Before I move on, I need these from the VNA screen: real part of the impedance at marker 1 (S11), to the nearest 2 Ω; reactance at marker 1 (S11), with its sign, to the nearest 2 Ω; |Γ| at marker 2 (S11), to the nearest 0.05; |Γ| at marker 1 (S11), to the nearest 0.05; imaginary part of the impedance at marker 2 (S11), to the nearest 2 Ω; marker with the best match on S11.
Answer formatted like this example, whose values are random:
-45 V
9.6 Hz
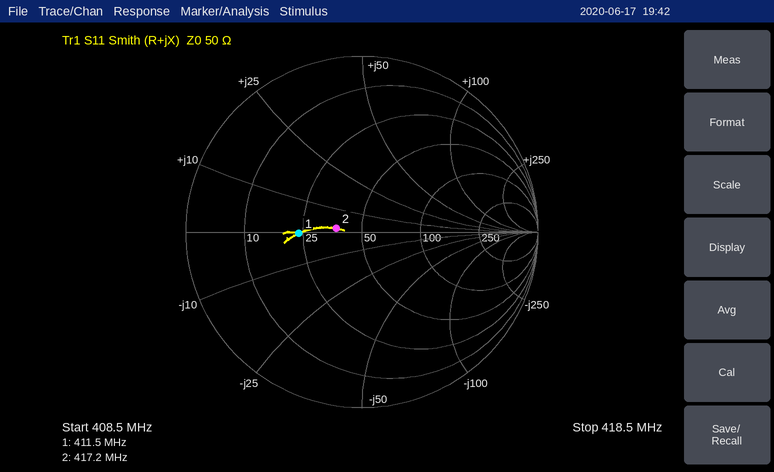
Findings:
24 Ω
0 Ω
0.15
0.35
+2 Ω
marker 2
